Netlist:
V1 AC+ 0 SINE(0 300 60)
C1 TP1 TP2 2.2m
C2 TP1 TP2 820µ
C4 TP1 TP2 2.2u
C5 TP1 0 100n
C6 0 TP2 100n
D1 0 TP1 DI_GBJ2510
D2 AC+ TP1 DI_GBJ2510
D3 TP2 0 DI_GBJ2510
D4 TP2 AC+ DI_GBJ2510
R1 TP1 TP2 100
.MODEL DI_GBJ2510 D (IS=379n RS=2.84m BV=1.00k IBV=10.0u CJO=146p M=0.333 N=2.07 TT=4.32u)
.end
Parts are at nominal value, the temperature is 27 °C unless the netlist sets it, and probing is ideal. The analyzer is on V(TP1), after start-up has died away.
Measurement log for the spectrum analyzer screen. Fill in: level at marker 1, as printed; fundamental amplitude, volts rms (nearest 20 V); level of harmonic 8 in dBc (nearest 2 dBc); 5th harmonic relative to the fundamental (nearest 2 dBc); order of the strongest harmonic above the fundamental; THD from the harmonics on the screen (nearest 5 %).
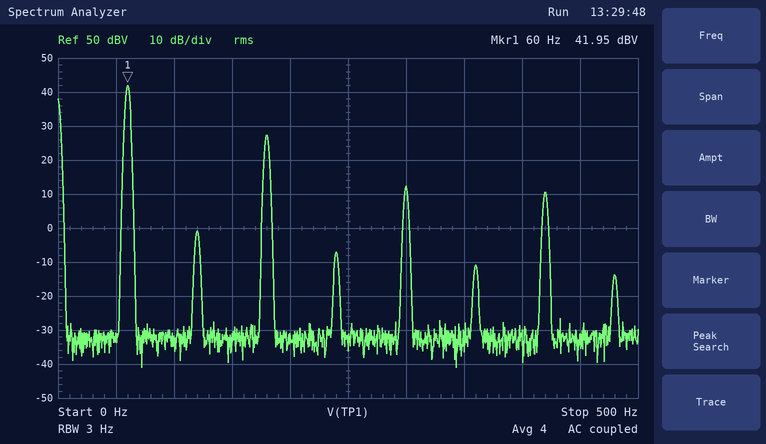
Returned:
41.95 dBV
120 V
-56 dBc
-30 dBc
3
20 %
